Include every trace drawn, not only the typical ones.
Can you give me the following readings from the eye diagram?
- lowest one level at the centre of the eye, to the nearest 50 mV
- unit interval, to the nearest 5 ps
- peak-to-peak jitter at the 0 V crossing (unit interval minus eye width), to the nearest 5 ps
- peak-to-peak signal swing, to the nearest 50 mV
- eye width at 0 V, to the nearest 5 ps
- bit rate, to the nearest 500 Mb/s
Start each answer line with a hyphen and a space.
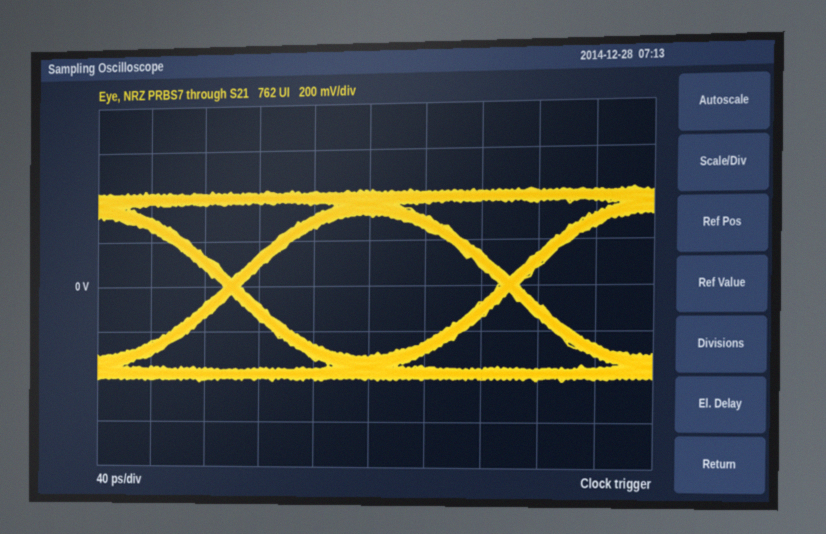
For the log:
- 300 mV
- 200 ps
- 15 ps
- 850 mV
- 185 ps
- 5.0 Gb/s
